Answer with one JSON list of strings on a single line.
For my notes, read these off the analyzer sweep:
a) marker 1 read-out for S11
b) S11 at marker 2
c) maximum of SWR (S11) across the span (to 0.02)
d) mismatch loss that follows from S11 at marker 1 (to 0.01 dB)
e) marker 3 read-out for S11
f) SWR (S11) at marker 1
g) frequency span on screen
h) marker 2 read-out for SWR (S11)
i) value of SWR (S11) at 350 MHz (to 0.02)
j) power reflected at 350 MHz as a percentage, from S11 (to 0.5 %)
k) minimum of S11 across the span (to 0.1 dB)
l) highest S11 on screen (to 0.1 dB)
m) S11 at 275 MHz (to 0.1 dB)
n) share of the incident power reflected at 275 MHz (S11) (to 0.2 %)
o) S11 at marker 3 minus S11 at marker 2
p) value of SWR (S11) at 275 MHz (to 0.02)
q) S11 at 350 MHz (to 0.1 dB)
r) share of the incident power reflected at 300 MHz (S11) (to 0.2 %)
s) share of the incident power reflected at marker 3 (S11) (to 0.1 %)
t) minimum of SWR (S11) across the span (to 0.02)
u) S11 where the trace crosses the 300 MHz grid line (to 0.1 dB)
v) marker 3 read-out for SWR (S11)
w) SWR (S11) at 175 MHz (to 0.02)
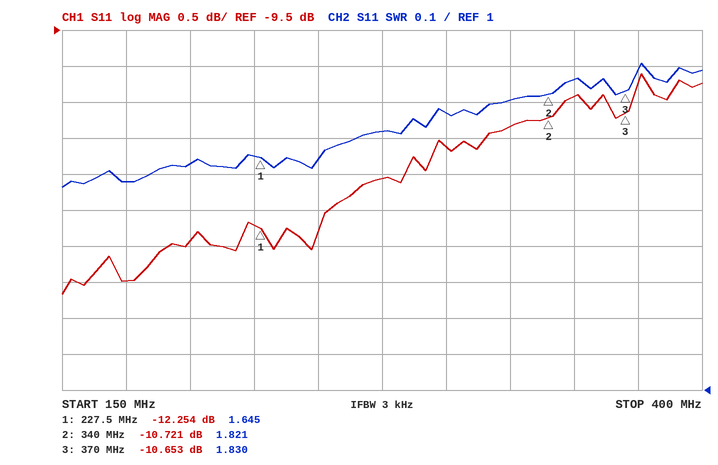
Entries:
["-12.254 dB", "-10.721 dB", "1.90", "0.27 dB", "-10.653 dB", "1.645", "250 MHz", "1.821", "1.86", "9.0 %", "-13.2 dB", "-10.1 dB", "-11.6 dB", "7.0 %", "0.068 dB", "1.72", "-10.4 dB", "7.8 %", "8.6 %", "1.56", "-11.1 dB", "1.830", "1.58"]
